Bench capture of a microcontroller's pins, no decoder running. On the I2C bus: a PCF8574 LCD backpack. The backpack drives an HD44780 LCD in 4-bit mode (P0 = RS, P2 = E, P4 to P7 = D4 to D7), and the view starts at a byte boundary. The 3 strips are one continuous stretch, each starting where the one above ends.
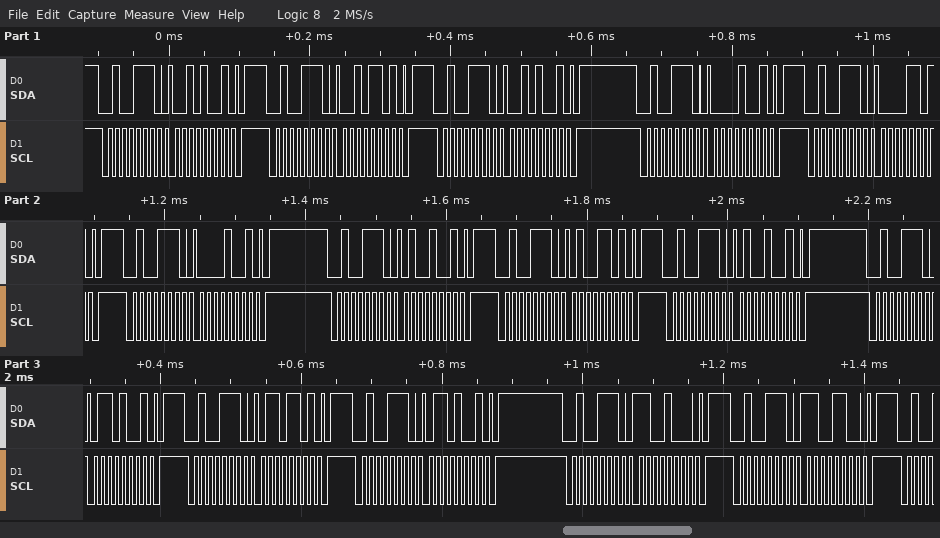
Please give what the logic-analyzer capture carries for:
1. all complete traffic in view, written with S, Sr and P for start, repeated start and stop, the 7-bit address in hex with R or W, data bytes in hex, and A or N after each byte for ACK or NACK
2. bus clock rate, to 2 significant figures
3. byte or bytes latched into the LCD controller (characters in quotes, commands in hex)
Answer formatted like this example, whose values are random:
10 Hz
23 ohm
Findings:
S 27W A 29 A P S 27W A 2D A P S 27W A 29 A P S 27W A 09 A P S 27W A 0D A P S 27W A 09 A P S 27W A 49 A P S 27W A 4D A P S 27W A 49 A P S 27W A 69 A P S 27W A 6D A P S 27W A 69 A P S 27W A C8 A P S 27W A CC A P
100 kHz
' ' 'F'
